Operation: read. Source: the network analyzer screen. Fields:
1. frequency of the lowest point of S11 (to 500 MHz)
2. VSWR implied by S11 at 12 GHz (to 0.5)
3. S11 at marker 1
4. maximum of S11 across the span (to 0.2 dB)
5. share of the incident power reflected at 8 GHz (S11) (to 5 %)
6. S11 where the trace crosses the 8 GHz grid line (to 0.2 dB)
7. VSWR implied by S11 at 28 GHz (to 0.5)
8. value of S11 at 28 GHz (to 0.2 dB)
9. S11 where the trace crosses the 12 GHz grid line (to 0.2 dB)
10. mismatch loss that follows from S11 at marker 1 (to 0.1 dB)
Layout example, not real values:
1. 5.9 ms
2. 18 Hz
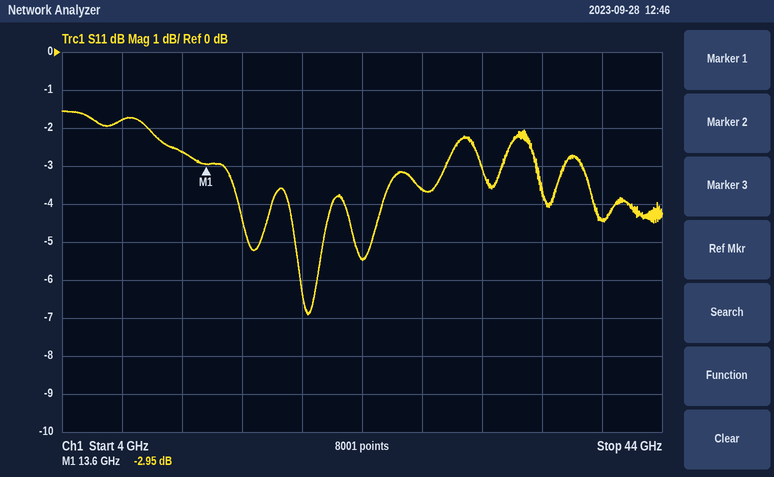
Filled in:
1. 20.5 GHz
2. 6.5
3. -2.95 dB
4. -1.6 dB
5. 65 %
6. -1.8 dB
7. 5.0
8. -3.6 dB
9. -2.6 dB
10. 3.1 dB
